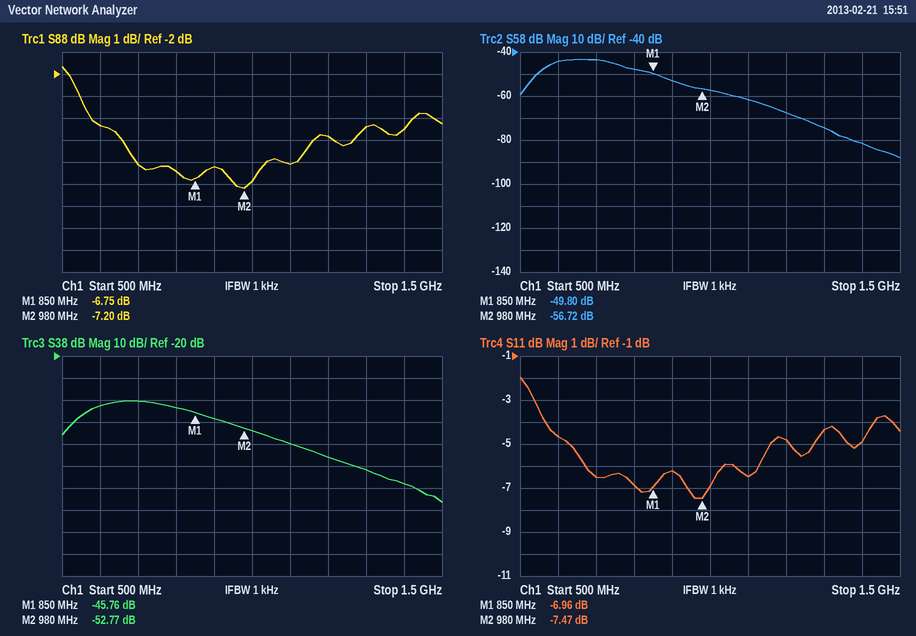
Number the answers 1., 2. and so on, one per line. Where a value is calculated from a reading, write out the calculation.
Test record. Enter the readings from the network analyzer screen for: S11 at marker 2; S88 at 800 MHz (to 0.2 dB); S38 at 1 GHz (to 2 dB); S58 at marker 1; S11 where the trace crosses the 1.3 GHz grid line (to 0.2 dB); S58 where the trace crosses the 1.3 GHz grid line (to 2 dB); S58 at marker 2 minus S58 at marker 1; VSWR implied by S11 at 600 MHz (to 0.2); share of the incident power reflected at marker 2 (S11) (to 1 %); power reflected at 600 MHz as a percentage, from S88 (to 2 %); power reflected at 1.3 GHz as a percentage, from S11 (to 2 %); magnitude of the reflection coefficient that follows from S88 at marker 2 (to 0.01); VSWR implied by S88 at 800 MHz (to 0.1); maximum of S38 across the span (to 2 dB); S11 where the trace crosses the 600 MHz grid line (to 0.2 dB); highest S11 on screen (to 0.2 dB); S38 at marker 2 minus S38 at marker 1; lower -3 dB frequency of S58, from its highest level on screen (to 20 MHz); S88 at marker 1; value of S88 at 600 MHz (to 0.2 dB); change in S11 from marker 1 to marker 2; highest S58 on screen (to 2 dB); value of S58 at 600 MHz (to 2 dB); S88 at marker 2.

1. -7.47 dB
2. -6.4 dB
3. -54 dB
4. -49.80 dB
5. -4.4 dB
6. -74 dB
7. -56.72 − (-49.8) = -6.92 dB
8. |Γ| = 10^(-4.6/20) = 0.5888; VSWR = (1 + 0.5888)/(1 − 0.5888) ≈ 3.86, so 3.8 to the nearest 0.2
9. 10^(-7.47/10) ≈ 18 %
10. 10^(-4.4/10) ≈ 36 %
11. 10^(-4.4/10) ≈ 36 %
12. 10^(-7.2/20) ≈ 0.44
13. |Γ| = 10^(-6.4/20) = 0.4786; VSWR = (1 + 0.4786)/(1 − 0.4786) ≈ 2.8
14. -40 dB
15. -4.6 dB
16. -2.0 dB
17. -52.77 − (-45.76) = -7.01 dB
18. 580 MHz
19. -6.75 dB
20. -4.4 dB
21. -7.47 − (-6.96) = -0.51 dB
22. -44 dB
23. -44 dB
24. -7.20 dB
